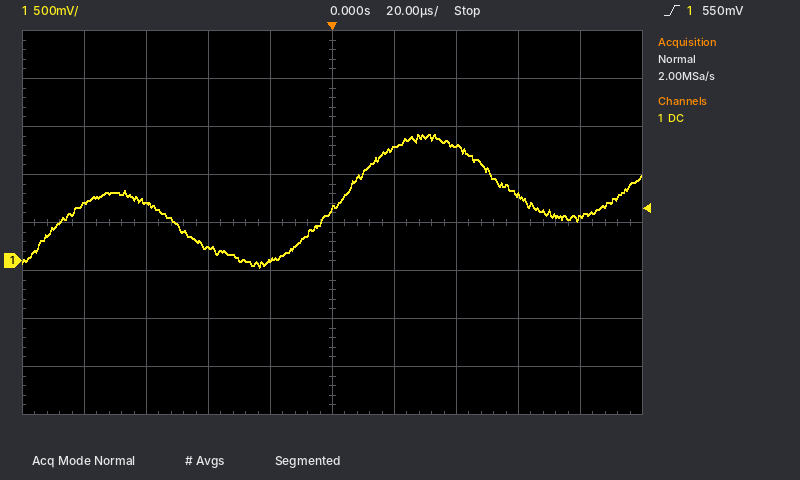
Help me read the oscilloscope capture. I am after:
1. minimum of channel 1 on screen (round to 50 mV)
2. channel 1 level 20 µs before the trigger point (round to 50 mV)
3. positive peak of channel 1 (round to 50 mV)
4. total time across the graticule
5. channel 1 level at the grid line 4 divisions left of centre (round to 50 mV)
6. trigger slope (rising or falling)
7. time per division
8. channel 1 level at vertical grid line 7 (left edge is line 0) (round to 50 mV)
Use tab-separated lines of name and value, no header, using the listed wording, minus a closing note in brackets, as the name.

minimum of channel 1 on screen	-50 mV
channel 1 level 20 µs before the trigger point	0 mV
positive peak of channel 1	1.30 V
total time across the graticule	200 µs
channel 1 level at the grid line 4 divisions left of centre	600 mV
trigger slope	rising
time per division	20 µs
channel 1 level at vertical grid line 7 (left edge is line 0)	1.20 V
